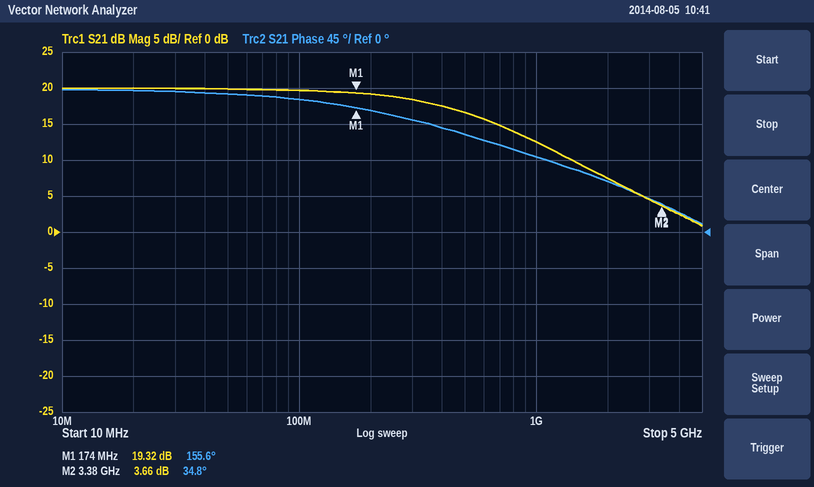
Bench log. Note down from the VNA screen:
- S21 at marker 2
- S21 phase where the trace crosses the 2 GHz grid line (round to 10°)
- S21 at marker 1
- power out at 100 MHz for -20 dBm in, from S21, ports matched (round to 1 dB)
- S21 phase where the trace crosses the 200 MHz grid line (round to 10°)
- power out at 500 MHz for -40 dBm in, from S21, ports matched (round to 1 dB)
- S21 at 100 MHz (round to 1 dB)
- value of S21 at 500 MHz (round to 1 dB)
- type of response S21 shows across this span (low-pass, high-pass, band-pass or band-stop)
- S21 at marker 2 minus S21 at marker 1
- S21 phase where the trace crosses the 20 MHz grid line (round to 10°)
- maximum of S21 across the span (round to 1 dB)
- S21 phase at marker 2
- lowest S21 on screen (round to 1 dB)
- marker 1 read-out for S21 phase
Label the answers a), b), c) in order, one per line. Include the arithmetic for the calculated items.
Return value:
a) 3.66 dB
b) 60°
c) 19.32 dB
d) -20 dBm + (20 dB) = 0 dBm
e) 150°
f) -40 dBm + (17 dB) = -23 dBm
g) 20 dB
h) 17 dB
i) low-pass
j) 3.66 − (19.32) = -15.66 dB
k) 180°
l) 20 dB
m) 34.8°
n) 1 dB
o) 155.6°
